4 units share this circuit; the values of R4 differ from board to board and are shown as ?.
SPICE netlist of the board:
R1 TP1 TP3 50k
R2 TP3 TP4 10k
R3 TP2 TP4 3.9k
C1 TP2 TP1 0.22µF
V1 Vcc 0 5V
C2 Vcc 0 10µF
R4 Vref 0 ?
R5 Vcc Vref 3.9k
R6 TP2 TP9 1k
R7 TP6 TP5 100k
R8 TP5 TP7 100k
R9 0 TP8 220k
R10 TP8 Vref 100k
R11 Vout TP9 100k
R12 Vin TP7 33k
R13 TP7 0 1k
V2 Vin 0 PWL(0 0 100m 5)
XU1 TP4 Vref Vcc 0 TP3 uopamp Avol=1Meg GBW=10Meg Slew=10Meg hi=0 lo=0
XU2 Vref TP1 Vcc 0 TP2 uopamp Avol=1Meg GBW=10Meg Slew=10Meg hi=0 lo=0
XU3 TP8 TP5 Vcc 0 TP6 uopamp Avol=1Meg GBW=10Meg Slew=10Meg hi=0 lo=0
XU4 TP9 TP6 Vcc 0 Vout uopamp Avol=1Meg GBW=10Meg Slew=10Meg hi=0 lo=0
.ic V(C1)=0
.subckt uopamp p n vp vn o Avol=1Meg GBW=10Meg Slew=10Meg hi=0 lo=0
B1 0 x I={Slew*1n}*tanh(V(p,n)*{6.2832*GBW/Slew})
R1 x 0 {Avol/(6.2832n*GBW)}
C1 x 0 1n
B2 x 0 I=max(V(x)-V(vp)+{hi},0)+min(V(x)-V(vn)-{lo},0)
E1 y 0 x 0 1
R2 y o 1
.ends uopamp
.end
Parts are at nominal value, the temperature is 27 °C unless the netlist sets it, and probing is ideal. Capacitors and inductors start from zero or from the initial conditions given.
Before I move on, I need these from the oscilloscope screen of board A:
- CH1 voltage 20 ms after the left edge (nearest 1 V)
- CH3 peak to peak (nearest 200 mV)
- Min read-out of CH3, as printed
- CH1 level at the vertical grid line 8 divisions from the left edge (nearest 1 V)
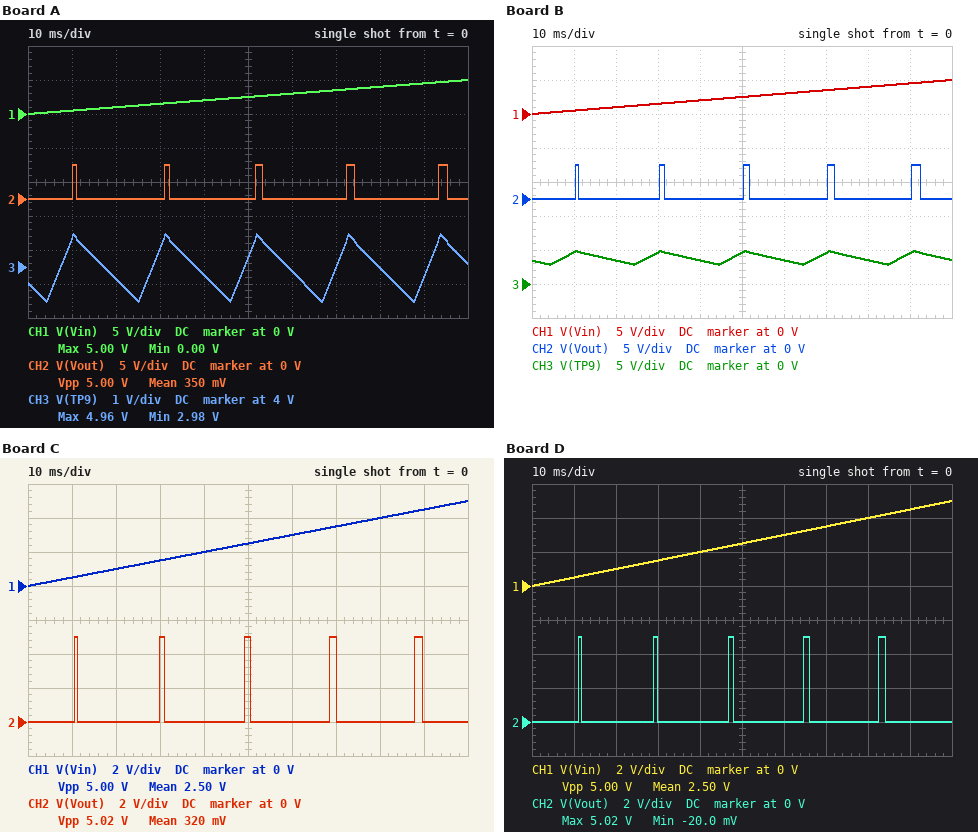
1 V
2.0 V
2.98 V
4 V
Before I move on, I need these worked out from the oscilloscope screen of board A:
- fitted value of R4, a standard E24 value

10 kΩ
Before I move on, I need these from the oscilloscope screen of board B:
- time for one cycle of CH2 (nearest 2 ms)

20 ms
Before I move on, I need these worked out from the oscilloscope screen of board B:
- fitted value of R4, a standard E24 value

9.1 kΩ
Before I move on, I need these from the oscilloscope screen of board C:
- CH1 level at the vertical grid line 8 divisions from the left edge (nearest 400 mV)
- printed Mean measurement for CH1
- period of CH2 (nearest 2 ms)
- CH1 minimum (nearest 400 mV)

4.0 V
2.50 V
20 ms
0 V
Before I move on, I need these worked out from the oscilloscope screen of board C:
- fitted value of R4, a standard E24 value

8.2 kΩ
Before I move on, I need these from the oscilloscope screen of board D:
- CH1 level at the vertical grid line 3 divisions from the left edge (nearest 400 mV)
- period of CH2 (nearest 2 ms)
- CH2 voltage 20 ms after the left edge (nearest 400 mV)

1.6 V
18 ms
0 V
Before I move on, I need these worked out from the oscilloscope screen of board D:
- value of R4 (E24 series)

6.2 kΩ
